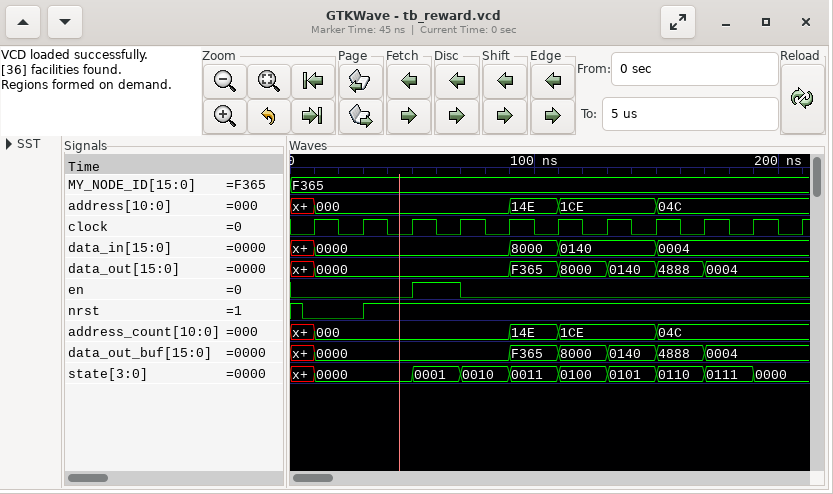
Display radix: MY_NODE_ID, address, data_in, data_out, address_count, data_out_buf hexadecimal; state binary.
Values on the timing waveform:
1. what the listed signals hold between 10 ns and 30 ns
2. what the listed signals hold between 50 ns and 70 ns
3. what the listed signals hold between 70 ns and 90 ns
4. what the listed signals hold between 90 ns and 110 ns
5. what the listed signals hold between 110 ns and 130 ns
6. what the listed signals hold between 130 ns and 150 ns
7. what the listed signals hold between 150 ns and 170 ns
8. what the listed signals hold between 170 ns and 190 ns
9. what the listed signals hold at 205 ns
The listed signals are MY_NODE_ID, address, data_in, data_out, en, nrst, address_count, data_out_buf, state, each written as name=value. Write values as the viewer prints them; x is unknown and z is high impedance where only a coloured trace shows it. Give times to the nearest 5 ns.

MY_NODE_ID=F365, address=000, data_in=0000, data_out=0000, en=0, nrst=0, address_count=000, data_out_buf=0000, state=0000
MY_NODE_ID=F365, address=000, data_in=0000, data_out=0000, en=1, nrst=1, address_count=000, data_out_buf=0000, state=0001
MY_NODE_ID=F365, address=000, data_in=0000, data_out=0000, en=0, nrst=1, address_count=000, data_out_buf=0000, state=0010
MY_NODE_ID=F365, address=14E, data_in=8000, data_out=F365, en=0, nrst=1, address_count=14E, data_out_buf=F365, state=0011
MY_NODE_ID=F365, address=1CE, data_in=0140, data_out=8000, en=0, nrst=1, address_count=1CE, data_out_buf=8000, state=0100
MY_NODE_ID=F365, address=1CE, data_in=0140, data_out=0140, en=0, nrst=1, address_count=1CE, data_out_buf=0140, state=0101
MY_NODE_ID=F365, address=04C, data_in=0004, data_out=4888, en=0, nrst=1, address_count=04C, data_out_buf=4888, state=0110
MY_NODE_ID=F365, address=04C, data_in=0004, data_out=0004, en=0, nrst=1, address_count=04C, data_out_buf=0004, state=0111
MY_NODE_ID=F365, address=04C, data_in=0004, data_out=0004, en=0, nrst=1, address_count=04C, data_out_buf=0004, state=0000
